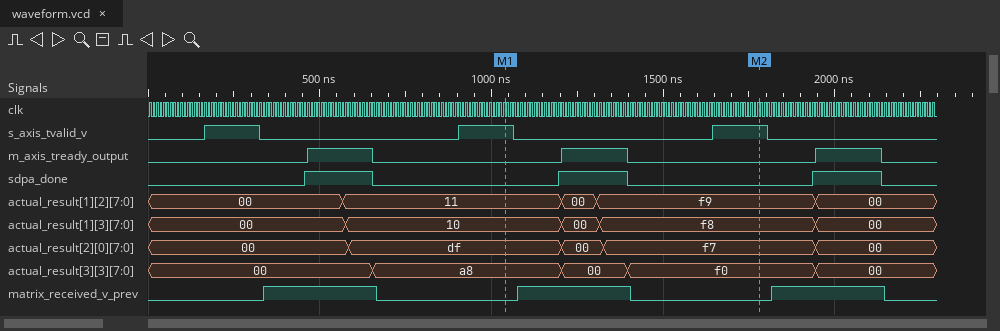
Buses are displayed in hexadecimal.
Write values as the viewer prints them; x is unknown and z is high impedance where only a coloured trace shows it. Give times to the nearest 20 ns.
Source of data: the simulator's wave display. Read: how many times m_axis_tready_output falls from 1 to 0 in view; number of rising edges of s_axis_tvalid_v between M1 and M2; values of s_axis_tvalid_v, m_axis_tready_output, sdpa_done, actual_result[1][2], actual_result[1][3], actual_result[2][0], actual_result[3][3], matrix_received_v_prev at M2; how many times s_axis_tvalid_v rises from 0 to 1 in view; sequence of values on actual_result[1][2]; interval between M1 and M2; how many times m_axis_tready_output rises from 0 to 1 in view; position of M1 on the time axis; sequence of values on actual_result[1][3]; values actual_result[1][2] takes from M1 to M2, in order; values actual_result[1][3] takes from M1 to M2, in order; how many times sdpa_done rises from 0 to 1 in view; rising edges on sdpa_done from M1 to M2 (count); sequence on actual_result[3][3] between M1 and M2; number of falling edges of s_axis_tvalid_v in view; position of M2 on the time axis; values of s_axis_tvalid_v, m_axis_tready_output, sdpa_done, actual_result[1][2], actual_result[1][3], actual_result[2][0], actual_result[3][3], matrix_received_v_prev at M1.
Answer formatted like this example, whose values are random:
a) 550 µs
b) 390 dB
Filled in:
a) 3
b) 1
c) s_axis_tvalid_v=1, m_axis_tready_output=0, sdpa_done=0, actual_result[1][2]=f9, actual_result[1][3]=f8, actual_result[2][0]=f7, actual_result[3][3]=f0, matrix_received_v_prev=0
d) 3
e) 00, 11, 00, f9, 00
f) 740 ns
g) 3
h) 1040 ns
i) 00, 10, 00, f8, 00
j) 11, 00, f9
k) 10, 00, f8
l) 3
m) 1
n) a8, 00, f0
o) 3
p) 1780 ns
q) s_axis_tvalid_v=1, m_axis_tready_output=0, sdpa_done=0, actual_result[1][2]=11, actual_result[1][3]=10, actual_result[2][0]=df, actual_result[3][3]=a8, matrix_received_v_prev=0
